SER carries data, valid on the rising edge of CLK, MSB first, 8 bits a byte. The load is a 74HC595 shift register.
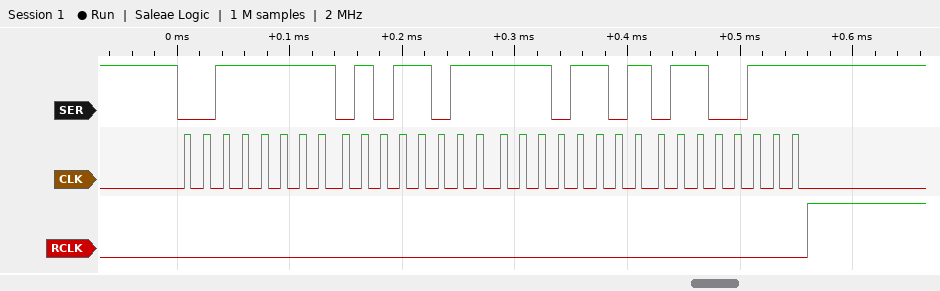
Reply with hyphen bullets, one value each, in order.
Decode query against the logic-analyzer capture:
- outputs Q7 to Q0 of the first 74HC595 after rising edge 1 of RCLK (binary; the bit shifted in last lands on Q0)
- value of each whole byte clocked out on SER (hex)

- 01100111
- 0x3F 0x5B 0xED 0x67
